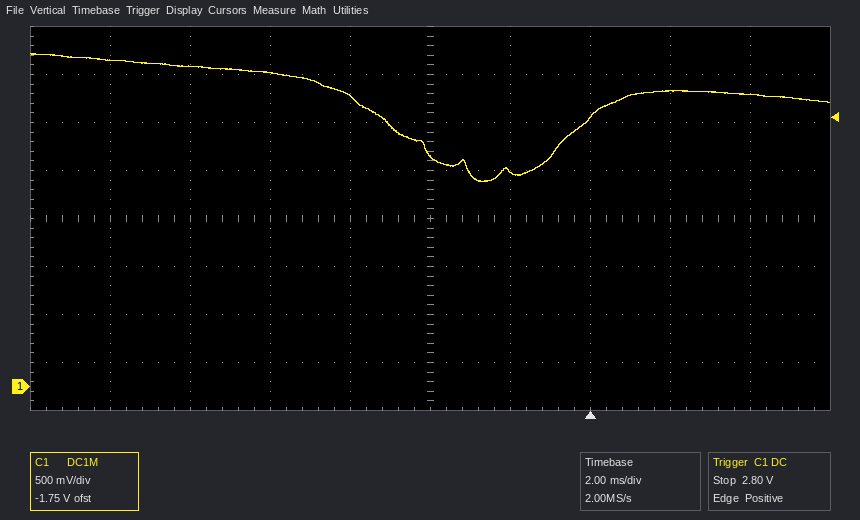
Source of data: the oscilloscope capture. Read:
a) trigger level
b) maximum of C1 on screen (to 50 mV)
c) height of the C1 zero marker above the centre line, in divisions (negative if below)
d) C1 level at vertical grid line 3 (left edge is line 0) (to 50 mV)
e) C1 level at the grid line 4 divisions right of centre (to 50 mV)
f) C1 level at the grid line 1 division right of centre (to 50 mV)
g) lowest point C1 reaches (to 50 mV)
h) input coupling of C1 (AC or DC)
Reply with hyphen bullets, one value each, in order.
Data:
- 2.80 V
- 3.45 V
- -3.5 div
- 3.25 V
- 3.05 V
- 2.25 V
- 2.15 V
- DC
